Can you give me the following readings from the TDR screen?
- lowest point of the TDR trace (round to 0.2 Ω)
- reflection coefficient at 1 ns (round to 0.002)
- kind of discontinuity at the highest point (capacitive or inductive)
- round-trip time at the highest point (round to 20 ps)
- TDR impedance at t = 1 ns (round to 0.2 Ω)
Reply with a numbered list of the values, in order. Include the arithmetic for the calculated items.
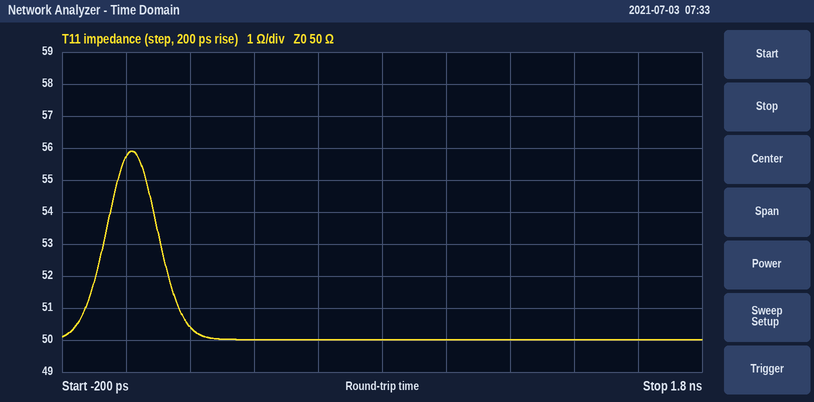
1. 50.0 Ω
2. (50 − 50)/(50 + 50) ≈ 0.000
3. inductive
4. 20 ps
5. 50.0 Ω
